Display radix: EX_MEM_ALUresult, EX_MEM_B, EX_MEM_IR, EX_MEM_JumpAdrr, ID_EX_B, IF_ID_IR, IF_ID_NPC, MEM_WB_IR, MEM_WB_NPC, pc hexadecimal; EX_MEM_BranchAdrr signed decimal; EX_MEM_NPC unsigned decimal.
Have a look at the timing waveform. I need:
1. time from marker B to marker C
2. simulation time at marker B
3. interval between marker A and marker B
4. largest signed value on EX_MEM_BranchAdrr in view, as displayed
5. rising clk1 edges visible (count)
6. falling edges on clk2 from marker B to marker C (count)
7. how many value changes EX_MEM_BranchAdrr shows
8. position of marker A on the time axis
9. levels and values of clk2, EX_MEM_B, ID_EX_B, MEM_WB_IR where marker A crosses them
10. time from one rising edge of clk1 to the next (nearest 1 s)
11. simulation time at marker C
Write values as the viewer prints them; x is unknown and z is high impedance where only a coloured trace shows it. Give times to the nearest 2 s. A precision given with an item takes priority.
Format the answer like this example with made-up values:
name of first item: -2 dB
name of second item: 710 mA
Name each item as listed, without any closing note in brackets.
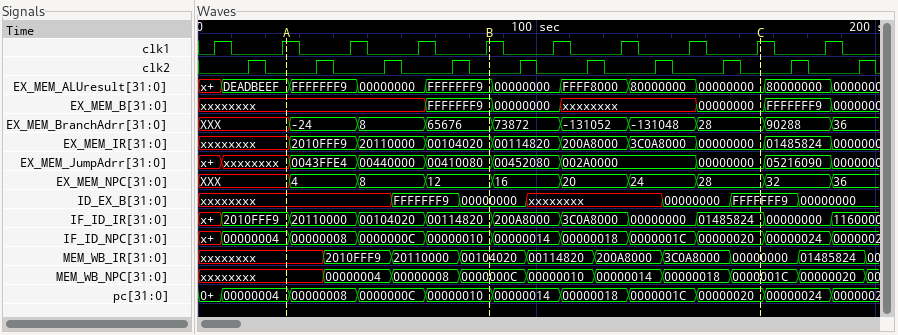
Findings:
time from marker B to marker C: 80 s
simulation time at marker B: 86 s
interval between marker A and marker B: 60 s
largest signed value on EX_MEM_BranchAdrr in view, as displayed: 90288
rising clk1 edges visible: 10
falling edges on clk2 from marker B to marker C: 4
how many value changes EX_MEM_BranchAdrr shows: 9
position of marker A on the time axis: 26 s
levels and values of clk2, EX_MEM_B, ID_EX_B, MEM_WB_IR where marker A crosses them: clk2=0, EX_MEM_B=xxxxxxxx, ID_EX_B=xxxxxxxx, MEM_WB_IR=xxxxxxxx
time from one rising edge of clk1 to the next: 20 s
simulation time at marker C: 166 s
